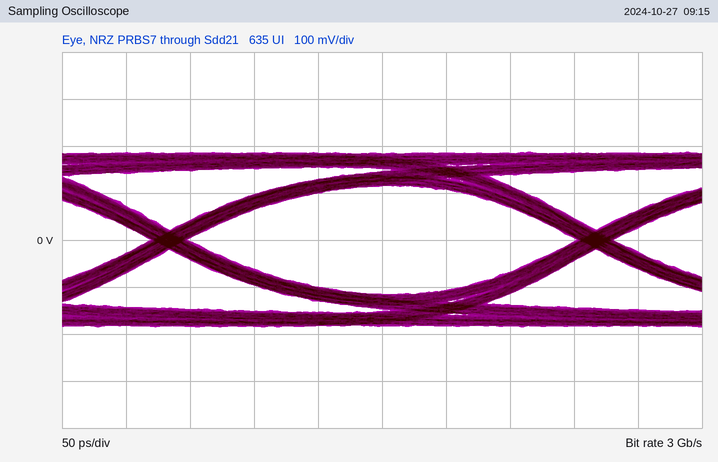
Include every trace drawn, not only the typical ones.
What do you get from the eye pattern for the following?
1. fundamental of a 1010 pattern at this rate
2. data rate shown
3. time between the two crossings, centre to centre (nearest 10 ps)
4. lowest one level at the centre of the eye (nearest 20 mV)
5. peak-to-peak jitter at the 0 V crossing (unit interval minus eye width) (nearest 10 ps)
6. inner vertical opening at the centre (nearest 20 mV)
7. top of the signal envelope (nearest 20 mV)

1.5 GHz
3 Gb/s
330 ps
120 mV
30 ps
240 mV
180 mV
